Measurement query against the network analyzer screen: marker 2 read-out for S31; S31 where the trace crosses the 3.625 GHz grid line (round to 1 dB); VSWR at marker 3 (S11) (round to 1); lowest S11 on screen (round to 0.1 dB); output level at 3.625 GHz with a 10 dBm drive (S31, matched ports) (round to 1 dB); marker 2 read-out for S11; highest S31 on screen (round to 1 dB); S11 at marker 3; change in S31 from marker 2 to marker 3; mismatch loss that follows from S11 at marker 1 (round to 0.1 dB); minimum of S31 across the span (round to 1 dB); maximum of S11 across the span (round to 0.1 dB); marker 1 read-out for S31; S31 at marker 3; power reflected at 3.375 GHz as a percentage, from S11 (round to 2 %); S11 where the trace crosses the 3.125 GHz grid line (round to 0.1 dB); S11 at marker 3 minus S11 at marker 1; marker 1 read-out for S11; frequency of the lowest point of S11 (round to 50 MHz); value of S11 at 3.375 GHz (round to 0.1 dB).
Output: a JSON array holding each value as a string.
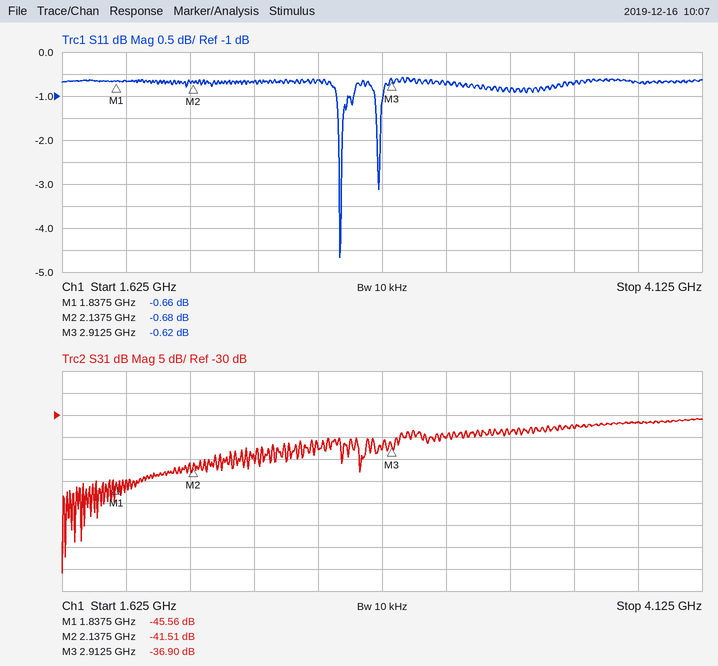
["-41.51 dB", "-33 dB", "28", "-4.7 dB", "-23 dBm", "-0.68 dB", "-31 dB", "-0.62 dB", "4.61 dB", "8.5 dB", "-66 dB", "-0.6 dB", "-45.56 dB", "-36.90 dB", "82 %", "-0.7 dB", "0.04 dB", "-0.66 dB", "2.70 GHz", "-0.9 dB"]
